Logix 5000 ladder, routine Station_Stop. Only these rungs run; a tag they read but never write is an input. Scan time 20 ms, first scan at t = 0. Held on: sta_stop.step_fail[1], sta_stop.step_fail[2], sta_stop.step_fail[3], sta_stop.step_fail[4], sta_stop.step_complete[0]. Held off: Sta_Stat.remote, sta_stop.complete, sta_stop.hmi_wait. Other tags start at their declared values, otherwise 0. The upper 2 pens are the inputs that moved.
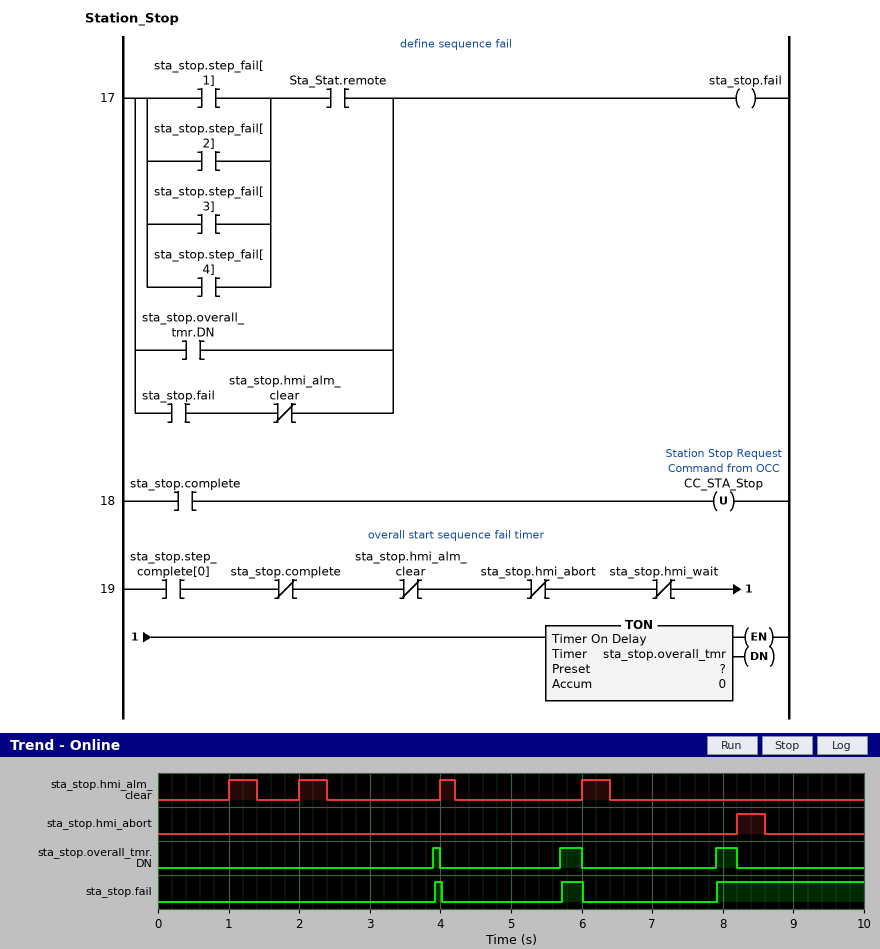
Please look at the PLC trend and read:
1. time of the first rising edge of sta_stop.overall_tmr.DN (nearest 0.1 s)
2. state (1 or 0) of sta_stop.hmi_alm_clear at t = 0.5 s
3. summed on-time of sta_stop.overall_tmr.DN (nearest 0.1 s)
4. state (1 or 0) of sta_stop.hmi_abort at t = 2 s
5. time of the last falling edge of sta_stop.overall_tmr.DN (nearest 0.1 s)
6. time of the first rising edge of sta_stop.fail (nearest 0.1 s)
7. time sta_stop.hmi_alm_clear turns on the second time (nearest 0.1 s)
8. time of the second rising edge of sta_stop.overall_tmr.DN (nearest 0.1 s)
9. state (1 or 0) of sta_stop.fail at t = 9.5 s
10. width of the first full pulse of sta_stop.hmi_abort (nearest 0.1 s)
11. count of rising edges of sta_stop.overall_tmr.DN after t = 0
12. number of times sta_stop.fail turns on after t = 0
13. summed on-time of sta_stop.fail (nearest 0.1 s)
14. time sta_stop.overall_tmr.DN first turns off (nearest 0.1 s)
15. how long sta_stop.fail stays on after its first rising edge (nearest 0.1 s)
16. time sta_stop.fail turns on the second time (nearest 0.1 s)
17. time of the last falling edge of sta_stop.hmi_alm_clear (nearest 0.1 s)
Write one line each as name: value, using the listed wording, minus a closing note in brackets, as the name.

time of the first rising edge of sta_stop.overall_tmr.DN: 3.9 s
state (1 or 0) of sta_stop.hmi_alm_clear at t = 0.5 s: 0
summed on-time of sta_stop.overall_tmr.DN: 0.7 s
state (1 or 0) of sta_stop.hmi_abort at t = 2 s: 0
time of the last falling edge of sta_stop.overall_tmr.DN: 8.2 s
time of the first rising edge of sta_stop.fail: 3.9 s
time sta_stop.hmi_alm_clear turns on the second time: 2.0 s
time of the second rising edge of sta_stop.overall_tmr.DN: 5.7 s
state (1 or 0) of sta_stop.fail at t = 9.5 s: 1
width of the first full pulse of sta_stop.hmi_abort: 0.4 s
count of rising edges of sta_stop.overall_tmr.DN after t = 0: 3
number of times sta_stop.fail turns on after t = 0: 3
summed on-time of sta_stop.fail: 2.5 s
time sta_stop.overall_tmr.DN first turns off: 4.0 s
how long sta_stop.fail stays on after its first rising edge: 0.1 s
time sta_stop.fail turns on the second time: 5.7 s
time of the last falling edge of sta_stop.hmi_alm_clear: 6.4 s
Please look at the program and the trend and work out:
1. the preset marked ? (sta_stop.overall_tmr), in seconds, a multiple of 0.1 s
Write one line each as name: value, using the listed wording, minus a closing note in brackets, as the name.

the preset marked ? (sta_stop.overall_tmr), in seconds, a multiple of 0.1 s: 1.5 s
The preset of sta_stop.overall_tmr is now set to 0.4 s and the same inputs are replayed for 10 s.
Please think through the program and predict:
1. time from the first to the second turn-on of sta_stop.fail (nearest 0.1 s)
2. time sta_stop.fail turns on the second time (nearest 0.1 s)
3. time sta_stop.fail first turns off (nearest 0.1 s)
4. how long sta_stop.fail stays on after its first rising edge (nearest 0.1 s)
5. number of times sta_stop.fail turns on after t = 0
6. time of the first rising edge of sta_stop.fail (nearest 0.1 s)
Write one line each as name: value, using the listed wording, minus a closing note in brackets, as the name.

time from the first to the second turn-on of sta_stop.fail: 1.4 s
time sta_stop.fail turns on the second time: 1.8 s
time sta_stop.fail first turns off: 1.0 s
how long sta_stop.fail stays on after its first rising edge: 0.6 s
number of times sta_stop.fail turns on after t = 0: 5
time of the first rising edge of sta_stop.fail: 0.4 s
